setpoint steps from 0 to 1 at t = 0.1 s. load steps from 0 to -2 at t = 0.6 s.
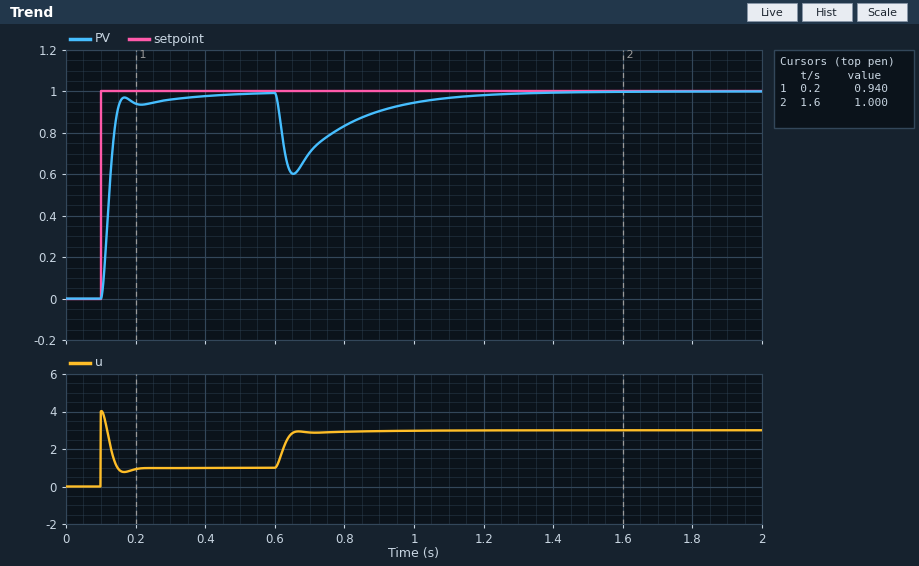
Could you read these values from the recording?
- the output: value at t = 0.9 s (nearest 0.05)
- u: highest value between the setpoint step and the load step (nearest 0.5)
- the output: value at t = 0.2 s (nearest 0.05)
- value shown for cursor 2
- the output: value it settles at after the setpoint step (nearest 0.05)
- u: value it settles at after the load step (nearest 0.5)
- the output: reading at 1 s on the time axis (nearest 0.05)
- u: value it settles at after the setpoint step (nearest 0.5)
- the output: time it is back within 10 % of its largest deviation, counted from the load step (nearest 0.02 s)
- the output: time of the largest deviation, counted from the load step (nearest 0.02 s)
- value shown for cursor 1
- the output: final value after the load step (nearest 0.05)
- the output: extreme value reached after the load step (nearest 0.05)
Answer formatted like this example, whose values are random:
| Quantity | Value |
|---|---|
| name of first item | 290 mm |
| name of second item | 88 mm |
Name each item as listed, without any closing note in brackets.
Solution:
| Quantity | Value |
|---|---|
| the output: value at t = 0.9 s | 0.90 |
| u: highest value between the setpoint step and the load step | 4.0 |
| the output: value at t = 0.2 s | 0.95 |
| value shown for cursor 2 | 1.000 |
| the output: value it settles at after the setpoint step | 1.00 |
| u: value it settles at after the load step | 3.0 |
| the output: reading at 1 s on the time axis | 0.95 |
| u: value it settles at after the setpoint step | 1.0 |
| the output: time it is back within 10 % of its largest deviation, counted from the load step | 0.46 s |
| the output: time of the largest deviation, counted from the load step | 0.06 s |
| value shown for cursor 1 | 0.940 |
| the output: final value after the load step | 1.00 |
| the output: extreme value reached after the load step | 0.60 |
